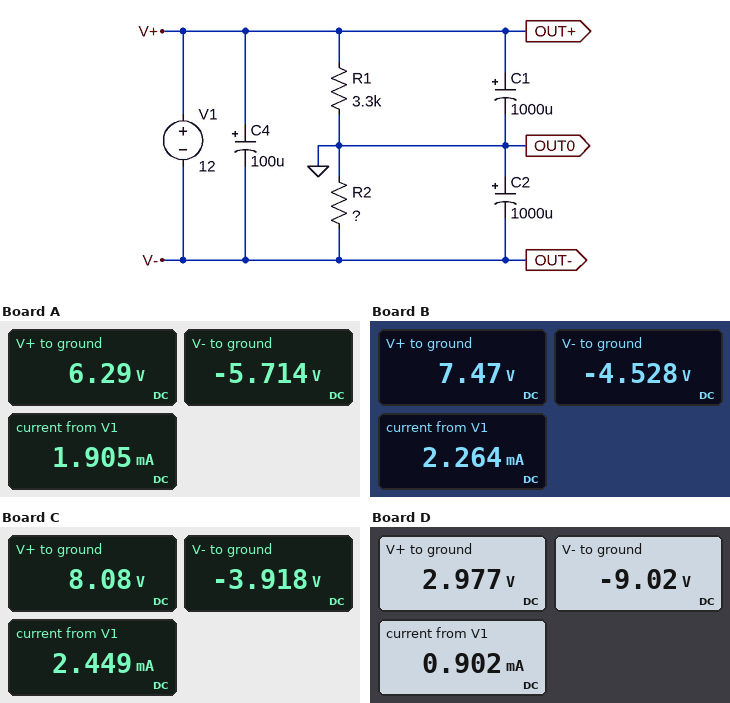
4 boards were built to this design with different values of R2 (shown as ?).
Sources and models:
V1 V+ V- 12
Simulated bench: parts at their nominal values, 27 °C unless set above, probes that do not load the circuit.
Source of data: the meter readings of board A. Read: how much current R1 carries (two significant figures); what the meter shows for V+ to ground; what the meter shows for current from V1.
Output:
1.9 mA
6.29 V
1.905 mA
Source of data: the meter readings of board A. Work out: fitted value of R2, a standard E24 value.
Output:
3 kΩ
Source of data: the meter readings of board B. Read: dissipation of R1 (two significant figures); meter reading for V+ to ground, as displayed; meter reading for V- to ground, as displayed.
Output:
17 mW
7.47 V
-4.528 V
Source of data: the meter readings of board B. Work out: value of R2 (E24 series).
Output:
2 kΩ
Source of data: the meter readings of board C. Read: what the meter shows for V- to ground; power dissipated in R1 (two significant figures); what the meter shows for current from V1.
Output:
-3.918 V
20 mW
2.449 mA
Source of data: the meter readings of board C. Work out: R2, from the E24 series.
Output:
1.6 kΩ
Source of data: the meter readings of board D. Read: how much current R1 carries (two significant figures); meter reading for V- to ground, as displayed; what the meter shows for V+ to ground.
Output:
900 µA
-9.02 V
2.977 V
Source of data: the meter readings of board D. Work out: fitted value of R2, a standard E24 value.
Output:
10 kΩ
